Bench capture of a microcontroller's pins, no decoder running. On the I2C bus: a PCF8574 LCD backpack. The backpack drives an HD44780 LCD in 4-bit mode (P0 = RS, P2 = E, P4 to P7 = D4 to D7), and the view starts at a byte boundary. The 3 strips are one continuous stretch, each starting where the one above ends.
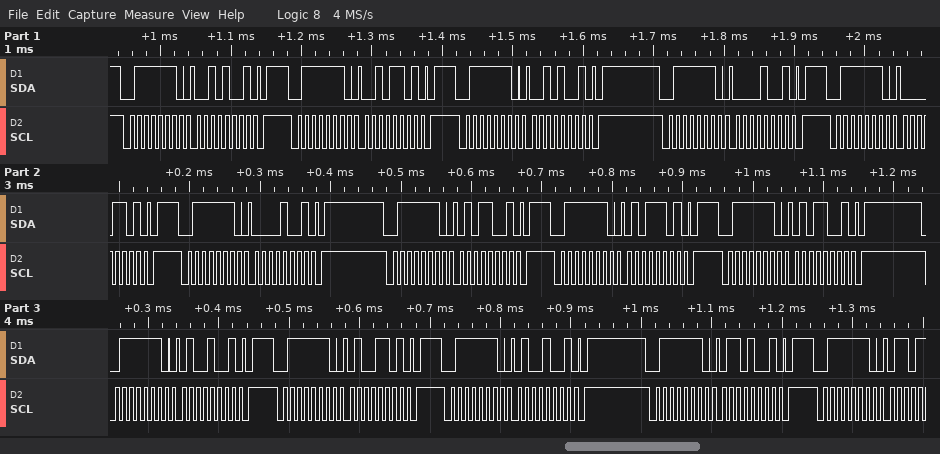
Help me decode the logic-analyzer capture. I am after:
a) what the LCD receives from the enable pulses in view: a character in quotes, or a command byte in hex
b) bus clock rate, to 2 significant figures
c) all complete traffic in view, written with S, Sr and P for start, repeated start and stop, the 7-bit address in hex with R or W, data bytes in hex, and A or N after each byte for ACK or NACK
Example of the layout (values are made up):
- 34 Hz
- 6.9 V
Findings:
- ' ' 'T'
- 100 kHz
- S 3FW A 29 A P S 3FW A 2D A P S 3FW A 29 A P S 3FW A 09 A P S 3FW A 0D A P S 3FW A 09 A P S 3FW A 59 A P S 3FW A 5D A P S 3FW A 59 A P S 3FW A 49 A P S 3FW A 4D A P S 3FW A 49 A P S 3FW A 69 A P S 3FW A
